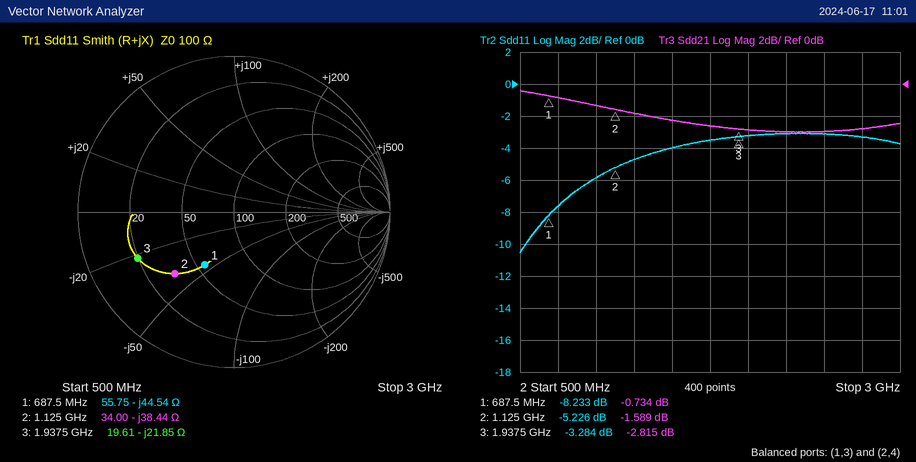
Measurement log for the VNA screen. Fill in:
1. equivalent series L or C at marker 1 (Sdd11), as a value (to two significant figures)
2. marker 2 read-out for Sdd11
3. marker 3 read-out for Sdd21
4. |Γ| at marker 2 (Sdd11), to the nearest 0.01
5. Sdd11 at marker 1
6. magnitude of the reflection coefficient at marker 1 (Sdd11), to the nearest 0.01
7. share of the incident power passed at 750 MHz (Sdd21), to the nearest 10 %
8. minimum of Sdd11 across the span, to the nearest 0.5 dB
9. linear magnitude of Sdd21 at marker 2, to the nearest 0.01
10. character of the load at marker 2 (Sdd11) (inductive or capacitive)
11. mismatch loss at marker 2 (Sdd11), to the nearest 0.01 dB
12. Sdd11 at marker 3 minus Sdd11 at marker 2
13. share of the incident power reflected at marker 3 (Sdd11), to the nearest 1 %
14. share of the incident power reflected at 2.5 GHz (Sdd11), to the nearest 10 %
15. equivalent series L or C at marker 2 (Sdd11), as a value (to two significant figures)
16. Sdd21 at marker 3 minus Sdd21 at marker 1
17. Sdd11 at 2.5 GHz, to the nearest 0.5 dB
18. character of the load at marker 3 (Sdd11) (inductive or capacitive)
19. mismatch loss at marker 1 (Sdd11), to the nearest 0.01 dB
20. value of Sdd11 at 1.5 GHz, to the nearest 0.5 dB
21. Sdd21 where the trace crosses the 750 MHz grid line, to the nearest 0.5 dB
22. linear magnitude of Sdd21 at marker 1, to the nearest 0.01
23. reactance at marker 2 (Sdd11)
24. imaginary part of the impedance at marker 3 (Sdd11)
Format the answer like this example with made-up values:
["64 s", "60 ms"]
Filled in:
["5.2 pF", "-5.226 dB", "-2.815 dB", "0.55", "-8.233 dB", "0.39", "80 %", "-10.5 dB", "0.83", "capacitive", "1.55 dB", "1.942 dB", "47 %", "50 %", "3.7 pF", "-2.081 dB", "-3.0 dB", "capacitive", "0.71 dB", "-4.0 dB", "-1.0 dB", "0.92", "-38.44 Ω", "-21.85 Ω"]
